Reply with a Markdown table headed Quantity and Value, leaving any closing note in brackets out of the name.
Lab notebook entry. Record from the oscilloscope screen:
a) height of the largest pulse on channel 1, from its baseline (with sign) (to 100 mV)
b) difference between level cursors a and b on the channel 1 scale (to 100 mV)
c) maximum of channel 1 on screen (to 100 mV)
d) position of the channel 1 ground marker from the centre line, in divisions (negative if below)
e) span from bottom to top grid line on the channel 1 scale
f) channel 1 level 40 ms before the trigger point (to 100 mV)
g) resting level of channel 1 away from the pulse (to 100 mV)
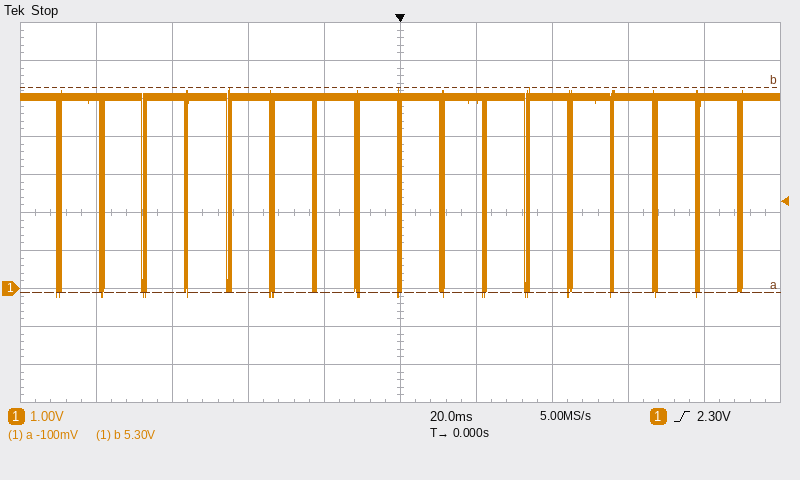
| Quantity | Value |
|---|---|
| height of the largest pulse on channel 1, from its baseline (with sign) | -5.3 V |
| difference between level cursors a and b on the channel 1 scale | 5.4 V |
| maximum of channel 1 on screen | 5.3 V |
| position of the channel 1 ground marker from the centre line, in divisions | -2.0 div |
| span from bottom to top grid line on the channel 1 scale | 10 V |
| channel 1 level 40 ms before the trigger point | 5.0 V |
| resting level of channel 1 away from the pulse | 5.0 V |
